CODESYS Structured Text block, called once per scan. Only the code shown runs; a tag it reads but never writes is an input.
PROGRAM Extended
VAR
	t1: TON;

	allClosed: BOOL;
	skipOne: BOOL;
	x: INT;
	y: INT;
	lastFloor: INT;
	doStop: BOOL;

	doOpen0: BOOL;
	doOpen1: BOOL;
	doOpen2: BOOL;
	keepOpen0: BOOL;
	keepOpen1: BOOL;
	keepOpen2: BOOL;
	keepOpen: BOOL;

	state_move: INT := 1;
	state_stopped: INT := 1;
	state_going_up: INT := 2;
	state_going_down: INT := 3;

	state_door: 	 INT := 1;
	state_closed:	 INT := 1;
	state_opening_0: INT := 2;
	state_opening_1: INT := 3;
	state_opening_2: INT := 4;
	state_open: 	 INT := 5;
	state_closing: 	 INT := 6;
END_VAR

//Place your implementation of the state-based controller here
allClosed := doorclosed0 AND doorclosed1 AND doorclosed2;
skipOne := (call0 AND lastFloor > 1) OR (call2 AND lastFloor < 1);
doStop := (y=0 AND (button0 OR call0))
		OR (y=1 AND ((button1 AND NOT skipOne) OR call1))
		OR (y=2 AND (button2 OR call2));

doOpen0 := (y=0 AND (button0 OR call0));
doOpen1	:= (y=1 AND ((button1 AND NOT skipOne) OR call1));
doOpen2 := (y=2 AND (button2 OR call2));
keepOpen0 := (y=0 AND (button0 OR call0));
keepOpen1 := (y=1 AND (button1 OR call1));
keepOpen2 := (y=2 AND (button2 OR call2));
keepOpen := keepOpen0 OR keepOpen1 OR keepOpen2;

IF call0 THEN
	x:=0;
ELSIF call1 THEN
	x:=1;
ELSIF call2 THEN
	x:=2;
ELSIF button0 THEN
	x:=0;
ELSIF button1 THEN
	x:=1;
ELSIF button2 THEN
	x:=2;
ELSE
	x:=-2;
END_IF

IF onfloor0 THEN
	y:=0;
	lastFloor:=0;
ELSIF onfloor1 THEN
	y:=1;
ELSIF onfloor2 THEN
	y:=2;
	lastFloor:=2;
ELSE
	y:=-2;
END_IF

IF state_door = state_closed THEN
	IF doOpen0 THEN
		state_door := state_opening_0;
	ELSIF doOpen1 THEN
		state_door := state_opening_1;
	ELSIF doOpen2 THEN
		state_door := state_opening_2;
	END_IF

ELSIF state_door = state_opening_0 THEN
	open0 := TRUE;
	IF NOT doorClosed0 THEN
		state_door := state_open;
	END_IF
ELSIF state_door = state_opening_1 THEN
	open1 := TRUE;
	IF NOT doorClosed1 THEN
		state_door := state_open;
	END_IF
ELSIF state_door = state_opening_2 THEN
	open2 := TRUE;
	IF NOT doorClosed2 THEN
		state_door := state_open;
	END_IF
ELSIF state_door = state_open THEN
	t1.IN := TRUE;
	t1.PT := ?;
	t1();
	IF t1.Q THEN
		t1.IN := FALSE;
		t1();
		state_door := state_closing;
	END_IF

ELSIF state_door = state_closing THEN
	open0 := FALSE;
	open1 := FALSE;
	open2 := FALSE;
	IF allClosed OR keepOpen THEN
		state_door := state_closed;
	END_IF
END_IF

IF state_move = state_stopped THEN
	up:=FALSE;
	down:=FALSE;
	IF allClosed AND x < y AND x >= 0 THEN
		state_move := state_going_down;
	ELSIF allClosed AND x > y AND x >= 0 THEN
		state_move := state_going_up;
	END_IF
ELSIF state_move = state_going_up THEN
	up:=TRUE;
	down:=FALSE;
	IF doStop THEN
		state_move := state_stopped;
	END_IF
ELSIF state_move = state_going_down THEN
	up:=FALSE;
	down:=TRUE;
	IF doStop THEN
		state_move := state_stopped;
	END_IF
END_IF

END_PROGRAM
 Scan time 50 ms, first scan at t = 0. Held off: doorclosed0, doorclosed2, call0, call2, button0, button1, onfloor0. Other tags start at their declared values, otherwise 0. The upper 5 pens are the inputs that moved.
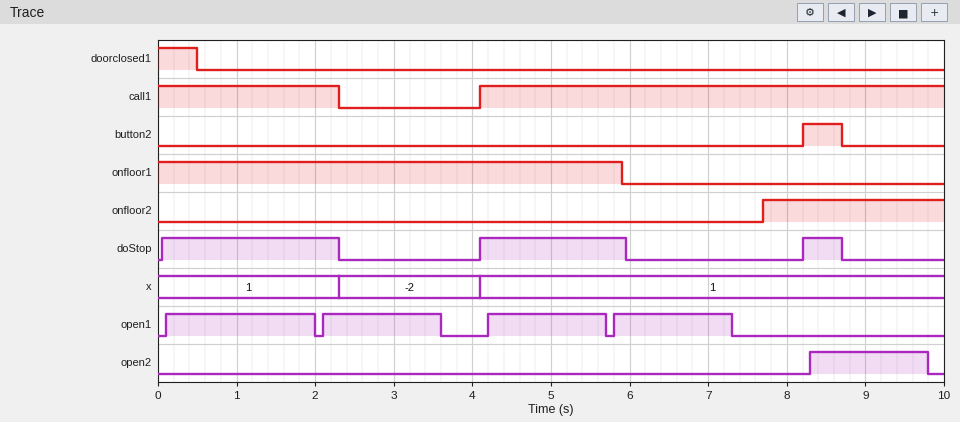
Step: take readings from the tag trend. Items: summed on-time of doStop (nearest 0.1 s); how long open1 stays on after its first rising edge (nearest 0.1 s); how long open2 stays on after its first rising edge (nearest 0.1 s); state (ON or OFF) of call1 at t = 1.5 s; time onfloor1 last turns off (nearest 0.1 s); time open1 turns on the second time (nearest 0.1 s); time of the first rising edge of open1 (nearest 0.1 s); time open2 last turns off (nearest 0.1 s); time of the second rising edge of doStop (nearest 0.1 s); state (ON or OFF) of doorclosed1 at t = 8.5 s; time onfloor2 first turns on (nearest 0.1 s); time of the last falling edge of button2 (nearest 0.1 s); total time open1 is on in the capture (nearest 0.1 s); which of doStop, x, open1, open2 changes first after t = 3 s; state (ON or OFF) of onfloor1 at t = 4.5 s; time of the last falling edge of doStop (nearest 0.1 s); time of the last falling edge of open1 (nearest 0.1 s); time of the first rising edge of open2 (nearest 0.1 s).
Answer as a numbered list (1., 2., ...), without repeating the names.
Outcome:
1. 4.6 s
2. 1.9 s
3. 1.5 s
4. ON
5. 5.9 s
6. 2.1 s
7. 0.1 s
8. 9.8 s
9. 4.1 s
10. OFF
11. 7.7 s
12. 8.7 s
13. 6.4 s
14. open1
15. ON
16. 8.7 s
17. 7.3 s
18. 8.3 s
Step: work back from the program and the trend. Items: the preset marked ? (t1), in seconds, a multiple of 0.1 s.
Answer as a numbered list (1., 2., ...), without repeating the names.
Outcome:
1. 1.4 s
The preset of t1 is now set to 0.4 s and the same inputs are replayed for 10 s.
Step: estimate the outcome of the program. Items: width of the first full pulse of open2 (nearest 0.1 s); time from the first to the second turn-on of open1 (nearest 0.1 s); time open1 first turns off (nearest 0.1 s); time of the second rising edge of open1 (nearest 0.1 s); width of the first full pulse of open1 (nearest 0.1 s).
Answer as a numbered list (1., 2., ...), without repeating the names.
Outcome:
1. 0.5 s
2. 1.0 s
3. 1.0 s
4. 1.1 s
5. 0.9 s
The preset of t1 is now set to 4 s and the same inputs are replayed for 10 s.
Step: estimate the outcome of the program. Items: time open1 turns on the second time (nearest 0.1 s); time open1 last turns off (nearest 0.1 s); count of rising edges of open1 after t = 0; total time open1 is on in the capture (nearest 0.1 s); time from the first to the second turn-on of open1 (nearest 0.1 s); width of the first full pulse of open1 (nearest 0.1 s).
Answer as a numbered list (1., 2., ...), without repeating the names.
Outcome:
1. 4.7 s
2. 8.8 s
3. 2
4. 8.6 s
5. 4.6 s
6. 4.5 s
